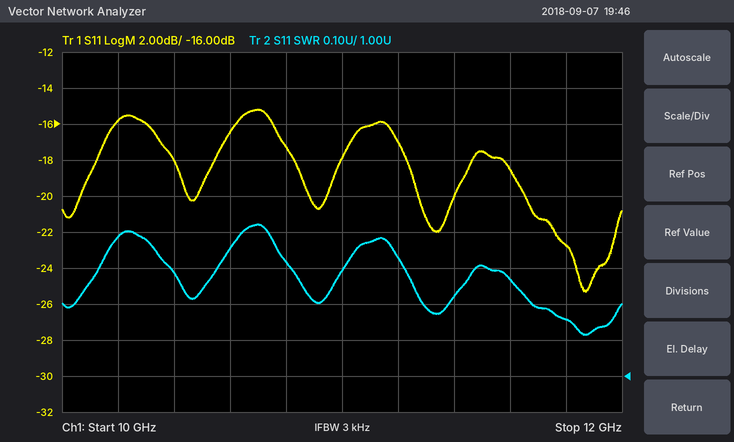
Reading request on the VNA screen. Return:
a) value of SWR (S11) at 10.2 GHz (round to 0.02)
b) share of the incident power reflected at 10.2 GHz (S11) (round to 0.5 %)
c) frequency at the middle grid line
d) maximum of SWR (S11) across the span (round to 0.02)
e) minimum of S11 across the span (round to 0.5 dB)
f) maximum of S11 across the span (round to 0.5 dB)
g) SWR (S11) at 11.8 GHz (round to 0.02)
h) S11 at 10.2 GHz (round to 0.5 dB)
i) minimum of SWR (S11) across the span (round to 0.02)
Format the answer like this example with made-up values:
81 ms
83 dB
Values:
1.38
2.5 %
11 GHz
1.42
-25.5 dB
-15.0 dB
1.16
-16.0 dB
1.12
